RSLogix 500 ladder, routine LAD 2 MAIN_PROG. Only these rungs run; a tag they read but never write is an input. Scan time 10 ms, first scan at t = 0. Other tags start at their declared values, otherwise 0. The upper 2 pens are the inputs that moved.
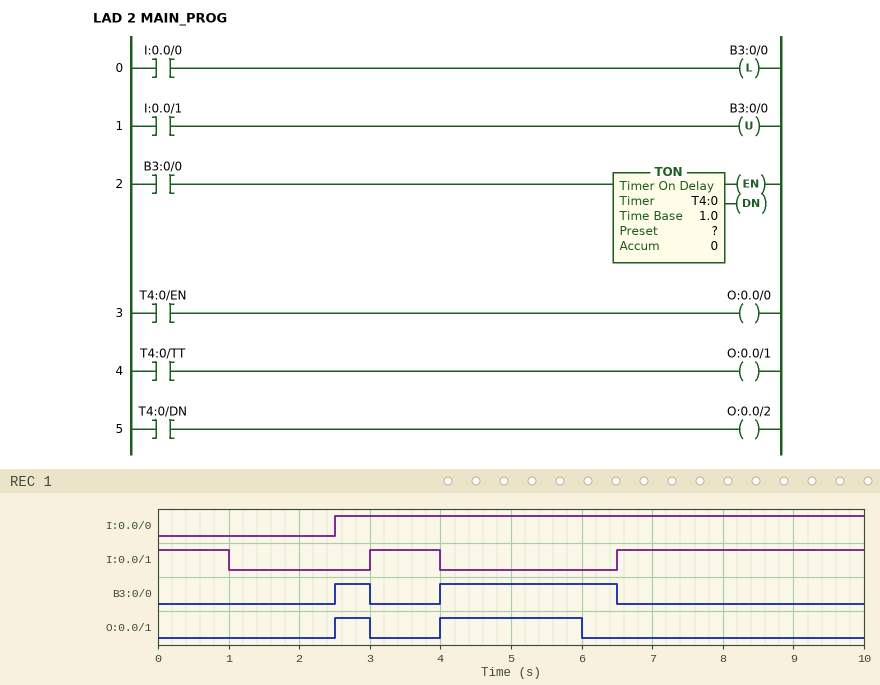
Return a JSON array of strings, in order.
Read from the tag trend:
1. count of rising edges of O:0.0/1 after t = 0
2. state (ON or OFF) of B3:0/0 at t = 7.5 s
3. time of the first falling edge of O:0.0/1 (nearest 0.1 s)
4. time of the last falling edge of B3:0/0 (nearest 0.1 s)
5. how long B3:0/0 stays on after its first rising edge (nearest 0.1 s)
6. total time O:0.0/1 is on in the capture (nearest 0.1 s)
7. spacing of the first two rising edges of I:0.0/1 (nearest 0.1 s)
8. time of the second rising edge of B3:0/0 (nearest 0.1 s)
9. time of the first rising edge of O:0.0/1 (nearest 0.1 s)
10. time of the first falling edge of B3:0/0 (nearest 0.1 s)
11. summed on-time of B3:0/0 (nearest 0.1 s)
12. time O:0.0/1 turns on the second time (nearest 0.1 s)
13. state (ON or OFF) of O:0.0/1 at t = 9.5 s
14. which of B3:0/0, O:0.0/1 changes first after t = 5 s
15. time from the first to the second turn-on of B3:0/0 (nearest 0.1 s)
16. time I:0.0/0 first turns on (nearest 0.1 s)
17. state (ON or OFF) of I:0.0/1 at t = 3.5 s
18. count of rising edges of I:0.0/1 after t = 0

["2", "OFF", "3.0 s", "6.5 s", "0.5 s", "2.5 s", "3.5 s", "4.0 s", "2.5 s", "3.0 s", "3.0 s", "4.0 s", "OFF", "O:0.0/1", "1.5 s", "2.5 s", "ON", "2"]
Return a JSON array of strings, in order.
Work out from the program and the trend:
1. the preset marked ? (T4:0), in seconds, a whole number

["2 s"]
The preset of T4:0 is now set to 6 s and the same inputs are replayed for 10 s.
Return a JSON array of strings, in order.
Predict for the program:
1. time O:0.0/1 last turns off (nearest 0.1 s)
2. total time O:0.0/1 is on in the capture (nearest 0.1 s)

["6.5 s", "3.0 s"]
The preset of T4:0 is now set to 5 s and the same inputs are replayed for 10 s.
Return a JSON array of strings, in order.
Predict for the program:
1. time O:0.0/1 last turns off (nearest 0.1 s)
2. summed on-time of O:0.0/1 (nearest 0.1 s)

["6.5 s", "3.0 s"]
